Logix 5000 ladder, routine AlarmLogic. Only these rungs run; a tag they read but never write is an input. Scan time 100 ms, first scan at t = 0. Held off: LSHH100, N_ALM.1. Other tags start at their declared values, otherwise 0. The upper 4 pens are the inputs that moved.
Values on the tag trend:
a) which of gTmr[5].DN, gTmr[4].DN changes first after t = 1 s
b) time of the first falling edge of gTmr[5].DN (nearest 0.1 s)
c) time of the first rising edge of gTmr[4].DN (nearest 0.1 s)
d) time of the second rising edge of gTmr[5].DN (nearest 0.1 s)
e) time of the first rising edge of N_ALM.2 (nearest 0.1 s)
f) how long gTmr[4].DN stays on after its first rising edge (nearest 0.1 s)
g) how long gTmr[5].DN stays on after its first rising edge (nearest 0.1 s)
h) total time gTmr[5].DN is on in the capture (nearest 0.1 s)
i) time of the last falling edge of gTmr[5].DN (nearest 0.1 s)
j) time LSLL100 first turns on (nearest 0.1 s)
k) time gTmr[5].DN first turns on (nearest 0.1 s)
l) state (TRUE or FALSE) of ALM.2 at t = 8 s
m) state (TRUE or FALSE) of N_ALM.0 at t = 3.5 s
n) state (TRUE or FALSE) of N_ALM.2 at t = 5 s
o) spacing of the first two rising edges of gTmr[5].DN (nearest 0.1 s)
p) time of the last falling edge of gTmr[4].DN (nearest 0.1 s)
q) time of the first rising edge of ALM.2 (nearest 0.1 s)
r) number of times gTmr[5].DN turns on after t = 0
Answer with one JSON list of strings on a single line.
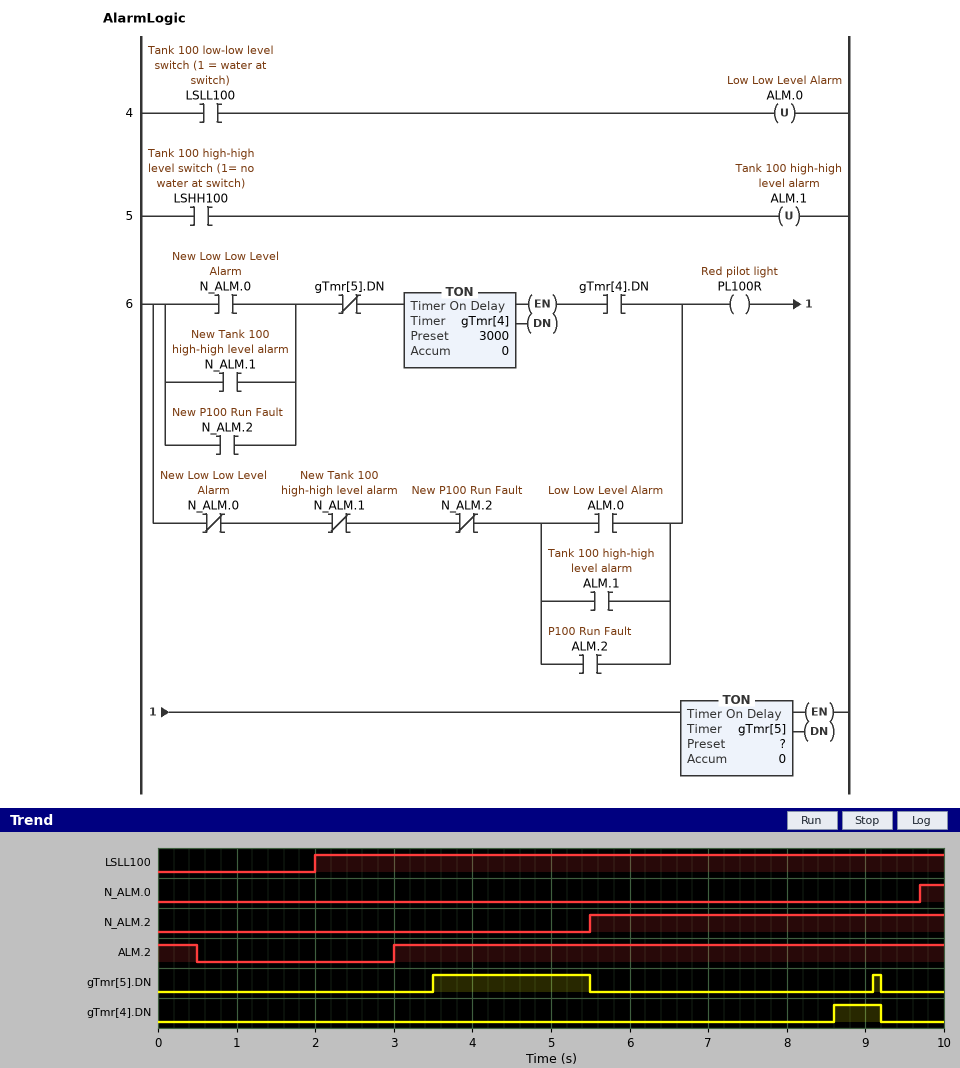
["gTmr[5].DN", "5.5 s", "8.6 s", "9.1 s", "5.5 s", "0.6 s", "2.0 s", "2.1 s", "9.2 s", "2.0 s", "3.5 s", "TRUE", "FALSE", "FALSE", "5.6 s", "9.2 s", "3.0 s", "2"]
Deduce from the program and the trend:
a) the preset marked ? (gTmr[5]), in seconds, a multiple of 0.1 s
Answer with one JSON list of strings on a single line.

["0.5 s"]
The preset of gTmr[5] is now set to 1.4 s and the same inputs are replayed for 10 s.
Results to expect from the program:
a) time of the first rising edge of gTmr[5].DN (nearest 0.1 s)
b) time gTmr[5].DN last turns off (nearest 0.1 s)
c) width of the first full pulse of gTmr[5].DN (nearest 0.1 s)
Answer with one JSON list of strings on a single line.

["4.4 s", "5.5 s", "1.1 s"]
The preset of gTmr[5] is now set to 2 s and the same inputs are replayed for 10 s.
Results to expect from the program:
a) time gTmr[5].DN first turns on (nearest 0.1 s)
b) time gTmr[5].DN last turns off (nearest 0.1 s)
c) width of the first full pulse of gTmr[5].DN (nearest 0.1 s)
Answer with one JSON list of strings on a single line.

["5.0 s", "5.5 s", "0.5 s"]
